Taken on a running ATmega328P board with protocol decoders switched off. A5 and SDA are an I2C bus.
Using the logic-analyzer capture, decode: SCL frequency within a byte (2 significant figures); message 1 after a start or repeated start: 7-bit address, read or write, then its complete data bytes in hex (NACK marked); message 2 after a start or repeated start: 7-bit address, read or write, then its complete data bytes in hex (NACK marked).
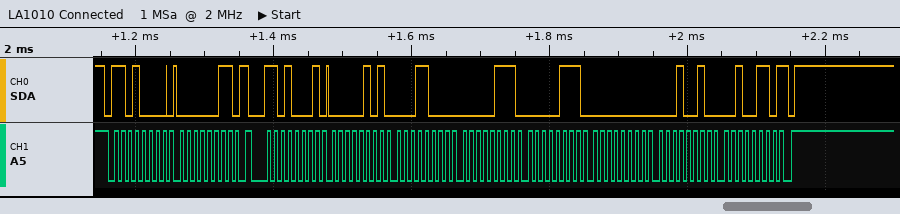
100 kHz
0x68 write: 03
0x68 read: 05 18 07 07 00 12 26 NACK
